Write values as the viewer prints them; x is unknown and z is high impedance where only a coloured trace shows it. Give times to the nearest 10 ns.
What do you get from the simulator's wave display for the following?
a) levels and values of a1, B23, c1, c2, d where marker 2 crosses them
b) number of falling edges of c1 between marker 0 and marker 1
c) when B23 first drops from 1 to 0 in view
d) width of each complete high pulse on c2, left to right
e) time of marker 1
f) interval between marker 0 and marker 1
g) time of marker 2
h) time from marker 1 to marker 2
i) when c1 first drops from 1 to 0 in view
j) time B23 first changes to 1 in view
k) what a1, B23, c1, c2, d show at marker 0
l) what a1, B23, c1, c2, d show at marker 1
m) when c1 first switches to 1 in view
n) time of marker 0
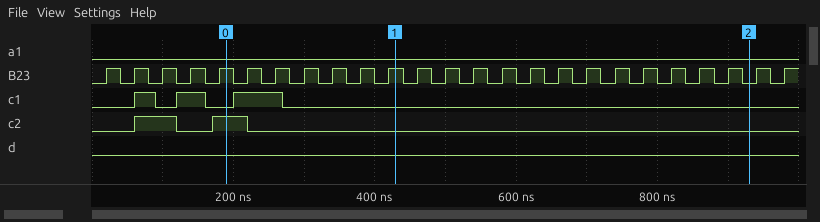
a1=0, B23=0, c1=0, c2=0, d=0
1
40 ns
60 ns, 50 ns
430 ns
240 ns
930 ns
500 ns
90 ns
20 ns
a1=0, B23=1, c1=0, c2=1, d=0
a1=0, B23=1, c1=0, c2=0, d=0
60 ns
190 ns
